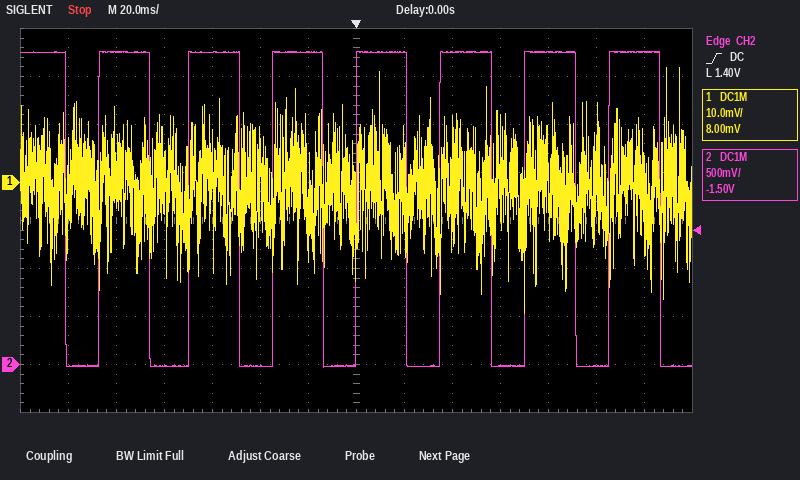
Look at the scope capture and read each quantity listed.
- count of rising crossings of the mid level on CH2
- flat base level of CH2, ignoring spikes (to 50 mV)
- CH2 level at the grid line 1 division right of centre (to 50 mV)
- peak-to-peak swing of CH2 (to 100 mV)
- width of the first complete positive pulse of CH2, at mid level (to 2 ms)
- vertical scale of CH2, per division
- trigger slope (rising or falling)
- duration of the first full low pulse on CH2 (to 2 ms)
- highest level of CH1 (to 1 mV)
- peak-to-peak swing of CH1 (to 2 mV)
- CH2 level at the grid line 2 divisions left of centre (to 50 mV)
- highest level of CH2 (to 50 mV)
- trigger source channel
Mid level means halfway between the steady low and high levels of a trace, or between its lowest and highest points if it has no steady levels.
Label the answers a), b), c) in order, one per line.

a) 7
b) 0 mV
c) 3.25 V
d) 3.30 V
e) 22 ms
f) 500 mV
g) rising
h) 14 ms
i) 24 mV
j) 52 mV
k) 0 mV
l) 3.25 V
m) CH2
